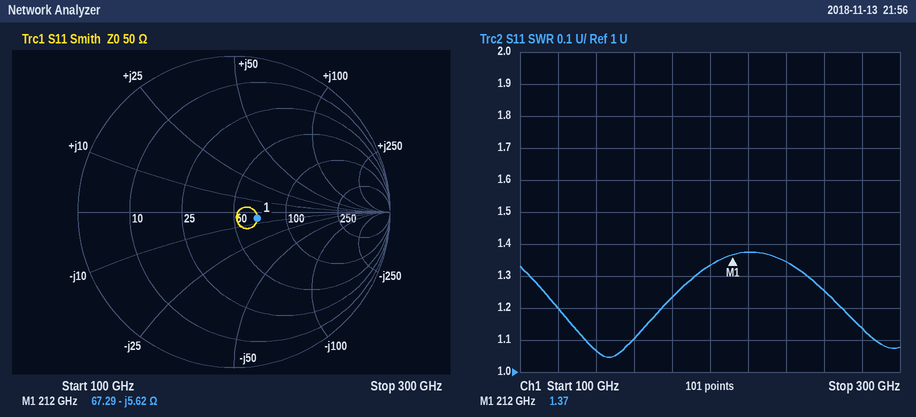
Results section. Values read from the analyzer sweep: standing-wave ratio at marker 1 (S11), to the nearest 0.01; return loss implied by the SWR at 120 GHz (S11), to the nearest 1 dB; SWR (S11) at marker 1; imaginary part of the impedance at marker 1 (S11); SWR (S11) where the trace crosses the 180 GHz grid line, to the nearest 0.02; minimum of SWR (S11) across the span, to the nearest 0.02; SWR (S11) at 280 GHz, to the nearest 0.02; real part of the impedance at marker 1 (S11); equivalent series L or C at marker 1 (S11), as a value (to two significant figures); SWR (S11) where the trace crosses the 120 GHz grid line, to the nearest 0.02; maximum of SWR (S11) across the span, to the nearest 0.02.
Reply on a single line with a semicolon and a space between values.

1.37; 21 dB; 1.37; -5.62 Ω; 1.24; 1.04; 1.14; 67.29 Ω; 130 fF; 1.20; 1.38
